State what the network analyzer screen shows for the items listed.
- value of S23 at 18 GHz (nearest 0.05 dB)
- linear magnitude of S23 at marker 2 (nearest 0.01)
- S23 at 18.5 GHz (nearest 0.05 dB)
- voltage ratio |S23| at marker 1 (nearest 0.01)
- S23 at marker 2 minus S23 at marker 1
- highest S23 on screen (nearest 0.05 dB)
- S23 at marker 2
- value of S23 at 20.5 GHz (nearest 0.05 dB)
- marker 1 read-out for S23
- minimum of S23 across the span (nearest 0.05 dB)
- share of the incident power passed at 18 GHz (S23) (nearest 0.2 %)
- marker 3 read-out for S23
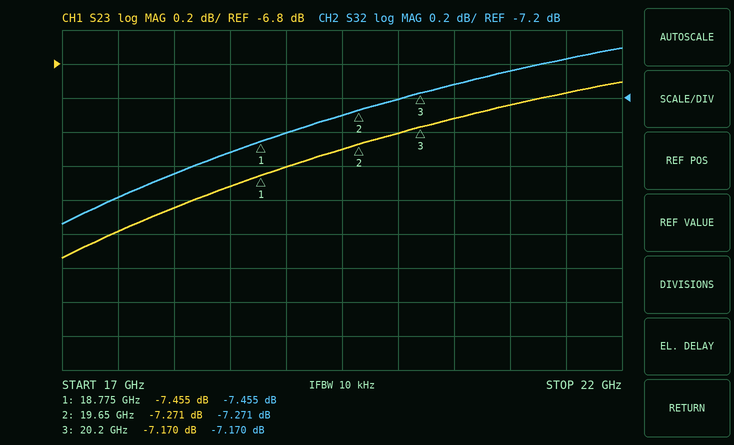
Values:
-7.65 dB
0.43
-7.50 dB
0.42
0.184 dB
-6.90 dB
-7.271 dB
-7.10 dB
-7.455 dB
-7.95 dB
17.2 %
-7.170 dB
